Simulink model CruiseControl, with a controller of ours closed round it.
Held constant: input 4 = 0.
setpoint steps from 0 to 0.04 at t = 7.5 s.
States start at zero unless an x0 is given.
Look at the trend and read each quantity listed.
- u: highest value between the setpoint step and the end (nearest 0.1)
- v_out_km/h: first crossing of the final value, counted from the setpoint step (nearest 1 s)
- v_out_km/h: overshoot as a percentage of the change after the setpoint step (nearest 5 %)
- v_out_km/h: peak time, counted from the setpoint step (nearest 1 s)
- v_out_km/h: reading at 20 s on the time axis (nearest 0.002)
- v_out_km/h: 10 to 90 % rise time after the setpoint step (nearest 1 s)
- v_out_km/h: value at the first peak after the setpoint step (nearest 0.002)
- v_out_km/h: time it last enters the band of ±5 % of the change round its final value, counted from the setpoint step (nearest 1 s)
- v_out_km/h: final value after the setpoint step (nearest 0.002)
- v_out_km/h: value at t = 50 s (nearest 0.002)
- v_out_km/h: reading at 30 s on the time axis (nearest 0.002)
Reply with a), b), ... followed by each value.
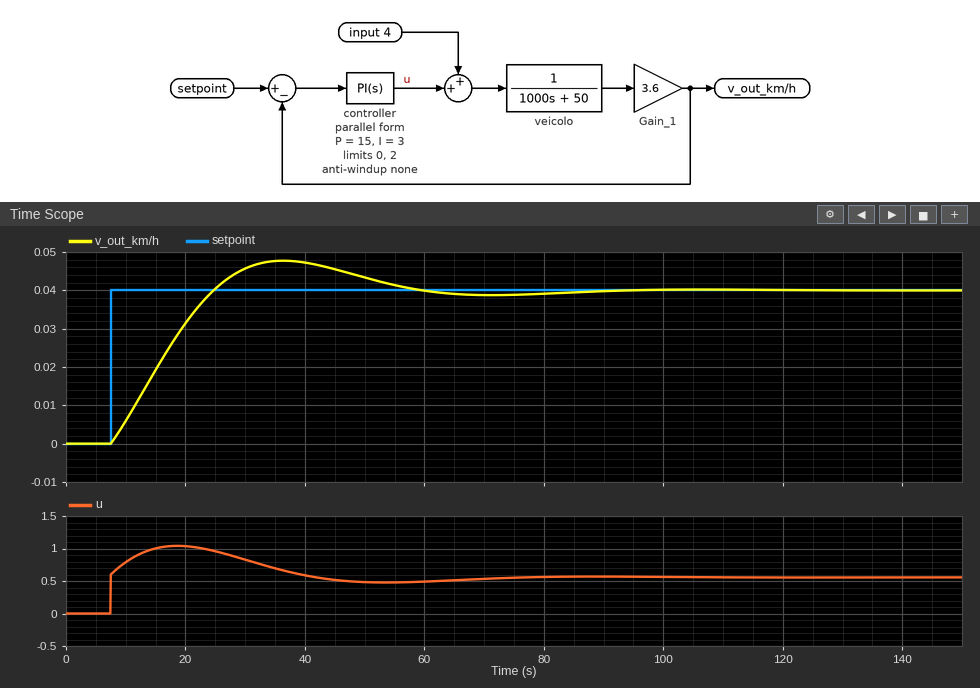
a) 1.0
b) 17 s
c) 20 %
d) 29 s
e) 0.032
f) 13 s
g) 0.048
h) 46 s
i) 0.040
j) 0.044
k) 0.046
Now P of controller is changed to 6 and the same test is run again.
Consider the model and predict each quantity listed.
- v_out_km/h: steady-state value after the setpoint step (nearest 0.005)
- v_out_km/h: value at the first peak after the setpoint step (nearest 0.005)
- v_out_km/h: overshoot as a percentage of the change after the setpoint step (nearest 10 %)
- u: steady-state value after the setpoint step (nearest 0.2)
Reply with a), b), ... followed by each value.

a) 0.040
b) 0.055
c) 30 %
d) 0.6
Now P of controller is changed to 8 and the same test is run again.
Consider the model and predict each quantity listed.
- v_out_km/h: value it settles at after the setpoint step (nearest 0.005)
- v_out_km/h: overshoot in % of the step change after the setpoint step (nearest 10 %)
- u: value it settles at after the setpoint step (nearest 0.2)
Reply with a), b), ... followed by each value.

a) 0.040
b) 30 %
c) 0.6
